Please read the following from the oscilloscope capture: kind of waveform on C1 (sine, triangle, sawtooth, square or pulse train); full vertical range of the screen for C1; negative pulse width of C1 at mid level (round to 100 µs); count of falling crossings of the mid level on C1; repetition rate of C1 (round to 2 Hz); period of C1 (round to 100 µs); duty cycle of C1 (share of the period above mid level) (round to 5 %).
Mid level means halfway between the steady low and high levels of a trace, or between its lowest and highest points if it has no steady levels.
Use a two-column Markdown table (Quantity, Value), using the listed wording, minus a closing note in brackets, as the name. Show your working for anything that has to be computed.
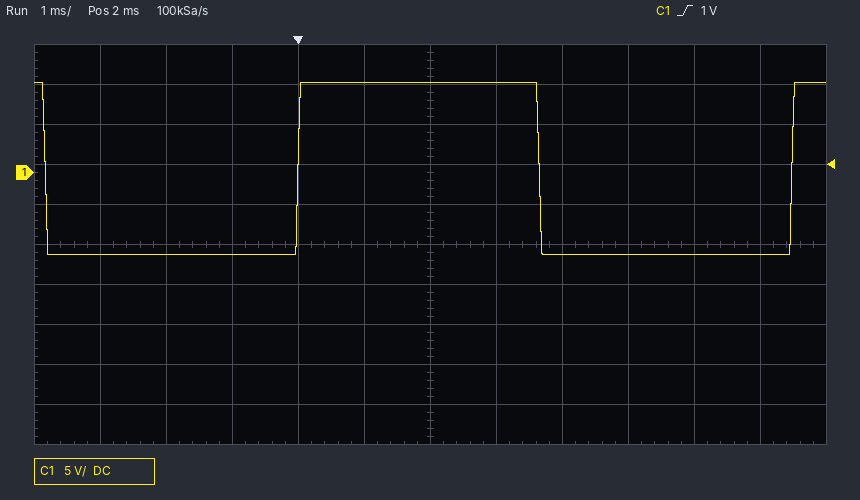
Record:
| Quantity | Value |
|---|---|
| kind of waveform on C1 | square |
| full vertical range of the screen for C1 | 50 V |
| negative pulse width of C1 at mid level | 3.8 ms |
| count of falling crossings of the mid level on C1 | 2 |
| repetition rate of C1 | 1 / 7.5 ms ≈ 133 Hz, so 134 Hz to the nearest 2 Hz |
| period of C1 | 7.5 ms |
| duty cycle of C1 (share of the period above mid level) | 50 % |
